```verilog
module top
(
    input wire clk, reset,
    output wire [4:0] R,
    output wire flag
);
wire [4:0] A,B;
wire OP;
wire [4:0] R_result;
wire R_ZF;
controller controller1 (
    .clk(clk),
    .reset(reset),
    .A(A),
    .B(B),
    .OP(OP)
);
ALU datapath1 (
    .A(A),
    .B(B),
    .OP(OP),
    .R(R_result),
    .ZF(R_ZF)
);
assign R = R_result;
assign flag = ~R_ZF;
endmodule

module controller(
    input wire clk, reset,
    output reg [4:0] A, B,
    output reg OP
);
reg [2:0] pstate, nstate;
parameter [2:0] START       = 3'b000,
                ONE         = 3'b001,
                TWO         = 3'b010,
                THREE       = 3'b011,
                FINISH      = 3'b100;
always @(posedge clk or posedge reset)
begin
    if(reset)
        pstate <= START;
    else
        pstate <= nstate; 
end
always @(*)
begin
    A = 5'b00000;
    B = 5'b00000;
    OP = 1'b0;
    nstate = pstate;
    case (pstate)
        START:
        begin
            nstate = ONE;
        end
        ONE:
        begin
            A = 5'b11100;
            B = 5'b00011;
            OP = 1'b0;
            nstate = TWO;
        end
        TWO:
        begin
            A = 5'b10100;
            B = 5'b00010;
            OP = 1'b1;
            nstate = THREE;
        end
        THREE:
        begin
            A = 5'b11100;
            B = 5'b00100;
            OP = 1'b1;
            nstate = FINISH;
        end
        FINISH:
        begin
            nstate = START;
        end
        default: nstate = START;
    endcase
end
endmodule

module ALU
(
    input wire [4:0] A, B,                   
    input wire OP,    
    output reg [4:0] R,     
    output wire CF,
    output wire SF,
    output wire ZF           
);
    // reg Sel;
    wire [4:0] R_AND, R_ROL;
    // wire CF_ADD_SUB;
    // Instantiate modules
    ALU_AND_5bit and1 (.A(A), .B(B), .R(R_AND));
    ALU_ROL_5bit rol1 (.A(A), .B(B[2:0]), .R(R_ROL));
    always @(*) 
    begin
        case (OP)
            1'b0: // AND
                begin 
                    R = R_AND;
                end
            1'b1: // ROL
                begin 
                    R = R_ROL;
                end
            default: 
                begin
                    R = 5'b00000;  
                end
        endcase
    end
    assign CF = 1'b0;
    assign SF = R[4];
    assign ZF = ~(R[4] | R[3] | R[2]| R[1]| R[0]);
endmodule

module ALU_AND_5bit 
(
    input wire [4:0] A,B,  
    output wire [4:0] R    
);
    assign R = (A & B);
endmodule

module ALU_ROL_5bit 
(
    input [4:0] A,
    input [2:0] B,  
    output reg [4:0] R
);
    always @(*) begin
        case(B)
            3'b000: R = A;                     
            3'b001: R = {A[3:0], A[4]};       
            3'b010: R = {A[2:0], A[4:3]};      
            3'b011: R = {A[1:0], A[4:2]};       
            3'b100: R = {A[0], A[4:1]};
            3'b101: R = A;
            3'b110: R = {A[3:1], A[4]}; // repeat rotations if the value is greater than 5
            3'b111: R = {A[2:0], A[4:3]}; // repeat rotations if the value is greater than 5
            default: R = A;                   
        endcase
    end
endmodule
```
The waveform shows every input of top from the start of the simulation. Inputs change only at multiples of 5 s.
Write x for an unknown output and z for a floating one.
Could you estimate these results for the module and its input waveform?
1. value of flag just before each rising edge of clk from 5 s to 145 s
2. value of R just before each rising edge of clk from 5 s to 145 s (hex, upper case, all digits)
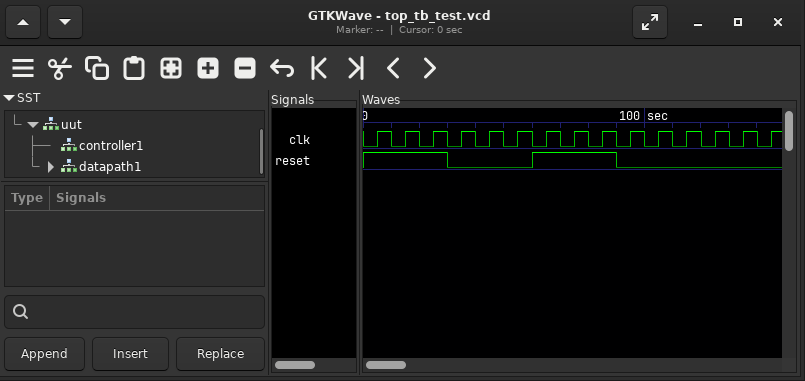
0 0 0 0 0 1 0 0 0 0 0 1 1 0 0
00, 00, 00, 00, 00, 12, 00, 00, 00, 00, 00, 12, 0E, 00, 00
